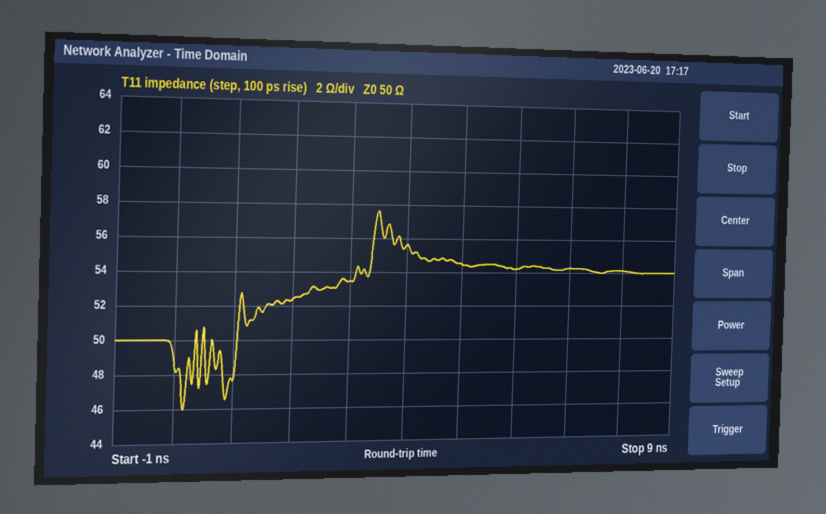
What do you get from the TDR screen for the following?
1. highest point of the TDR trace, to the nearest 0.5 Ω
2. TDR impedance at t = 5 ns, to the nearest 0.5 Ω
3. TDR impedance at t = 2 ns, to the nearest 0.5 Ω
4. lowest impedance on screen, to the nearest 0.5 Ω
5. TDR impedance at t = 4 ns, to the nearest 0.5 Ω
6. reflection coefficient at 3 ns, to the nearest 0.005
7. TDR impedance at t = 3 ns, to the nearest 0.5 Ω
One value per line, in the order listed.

57.5 Ω
54.5 Ω
52.5 Ω
46.0 Ω
55.5 Ω
+0.035
53.5 Ω
